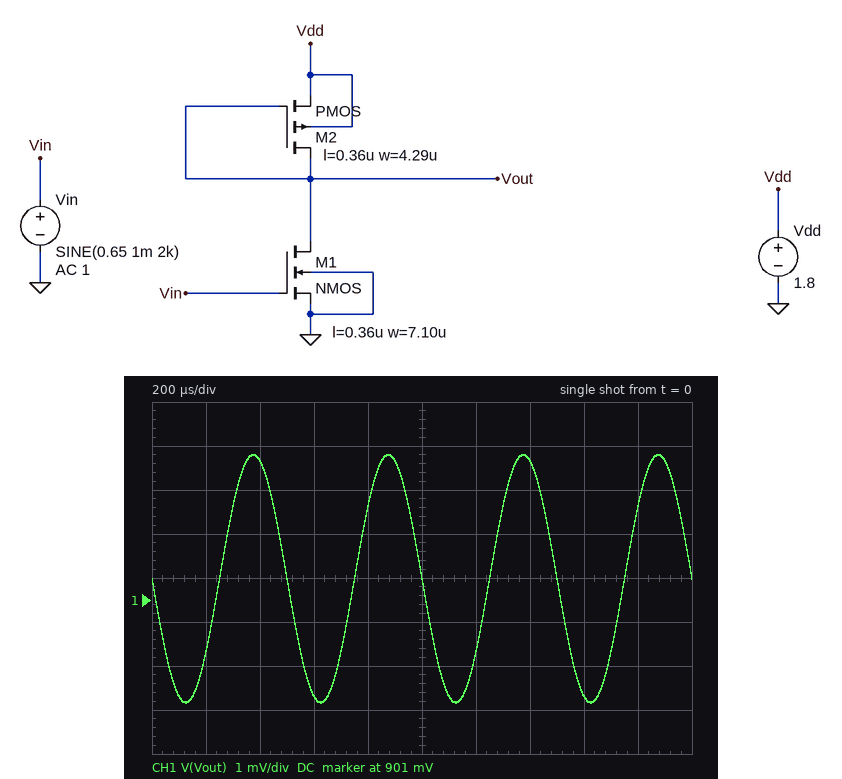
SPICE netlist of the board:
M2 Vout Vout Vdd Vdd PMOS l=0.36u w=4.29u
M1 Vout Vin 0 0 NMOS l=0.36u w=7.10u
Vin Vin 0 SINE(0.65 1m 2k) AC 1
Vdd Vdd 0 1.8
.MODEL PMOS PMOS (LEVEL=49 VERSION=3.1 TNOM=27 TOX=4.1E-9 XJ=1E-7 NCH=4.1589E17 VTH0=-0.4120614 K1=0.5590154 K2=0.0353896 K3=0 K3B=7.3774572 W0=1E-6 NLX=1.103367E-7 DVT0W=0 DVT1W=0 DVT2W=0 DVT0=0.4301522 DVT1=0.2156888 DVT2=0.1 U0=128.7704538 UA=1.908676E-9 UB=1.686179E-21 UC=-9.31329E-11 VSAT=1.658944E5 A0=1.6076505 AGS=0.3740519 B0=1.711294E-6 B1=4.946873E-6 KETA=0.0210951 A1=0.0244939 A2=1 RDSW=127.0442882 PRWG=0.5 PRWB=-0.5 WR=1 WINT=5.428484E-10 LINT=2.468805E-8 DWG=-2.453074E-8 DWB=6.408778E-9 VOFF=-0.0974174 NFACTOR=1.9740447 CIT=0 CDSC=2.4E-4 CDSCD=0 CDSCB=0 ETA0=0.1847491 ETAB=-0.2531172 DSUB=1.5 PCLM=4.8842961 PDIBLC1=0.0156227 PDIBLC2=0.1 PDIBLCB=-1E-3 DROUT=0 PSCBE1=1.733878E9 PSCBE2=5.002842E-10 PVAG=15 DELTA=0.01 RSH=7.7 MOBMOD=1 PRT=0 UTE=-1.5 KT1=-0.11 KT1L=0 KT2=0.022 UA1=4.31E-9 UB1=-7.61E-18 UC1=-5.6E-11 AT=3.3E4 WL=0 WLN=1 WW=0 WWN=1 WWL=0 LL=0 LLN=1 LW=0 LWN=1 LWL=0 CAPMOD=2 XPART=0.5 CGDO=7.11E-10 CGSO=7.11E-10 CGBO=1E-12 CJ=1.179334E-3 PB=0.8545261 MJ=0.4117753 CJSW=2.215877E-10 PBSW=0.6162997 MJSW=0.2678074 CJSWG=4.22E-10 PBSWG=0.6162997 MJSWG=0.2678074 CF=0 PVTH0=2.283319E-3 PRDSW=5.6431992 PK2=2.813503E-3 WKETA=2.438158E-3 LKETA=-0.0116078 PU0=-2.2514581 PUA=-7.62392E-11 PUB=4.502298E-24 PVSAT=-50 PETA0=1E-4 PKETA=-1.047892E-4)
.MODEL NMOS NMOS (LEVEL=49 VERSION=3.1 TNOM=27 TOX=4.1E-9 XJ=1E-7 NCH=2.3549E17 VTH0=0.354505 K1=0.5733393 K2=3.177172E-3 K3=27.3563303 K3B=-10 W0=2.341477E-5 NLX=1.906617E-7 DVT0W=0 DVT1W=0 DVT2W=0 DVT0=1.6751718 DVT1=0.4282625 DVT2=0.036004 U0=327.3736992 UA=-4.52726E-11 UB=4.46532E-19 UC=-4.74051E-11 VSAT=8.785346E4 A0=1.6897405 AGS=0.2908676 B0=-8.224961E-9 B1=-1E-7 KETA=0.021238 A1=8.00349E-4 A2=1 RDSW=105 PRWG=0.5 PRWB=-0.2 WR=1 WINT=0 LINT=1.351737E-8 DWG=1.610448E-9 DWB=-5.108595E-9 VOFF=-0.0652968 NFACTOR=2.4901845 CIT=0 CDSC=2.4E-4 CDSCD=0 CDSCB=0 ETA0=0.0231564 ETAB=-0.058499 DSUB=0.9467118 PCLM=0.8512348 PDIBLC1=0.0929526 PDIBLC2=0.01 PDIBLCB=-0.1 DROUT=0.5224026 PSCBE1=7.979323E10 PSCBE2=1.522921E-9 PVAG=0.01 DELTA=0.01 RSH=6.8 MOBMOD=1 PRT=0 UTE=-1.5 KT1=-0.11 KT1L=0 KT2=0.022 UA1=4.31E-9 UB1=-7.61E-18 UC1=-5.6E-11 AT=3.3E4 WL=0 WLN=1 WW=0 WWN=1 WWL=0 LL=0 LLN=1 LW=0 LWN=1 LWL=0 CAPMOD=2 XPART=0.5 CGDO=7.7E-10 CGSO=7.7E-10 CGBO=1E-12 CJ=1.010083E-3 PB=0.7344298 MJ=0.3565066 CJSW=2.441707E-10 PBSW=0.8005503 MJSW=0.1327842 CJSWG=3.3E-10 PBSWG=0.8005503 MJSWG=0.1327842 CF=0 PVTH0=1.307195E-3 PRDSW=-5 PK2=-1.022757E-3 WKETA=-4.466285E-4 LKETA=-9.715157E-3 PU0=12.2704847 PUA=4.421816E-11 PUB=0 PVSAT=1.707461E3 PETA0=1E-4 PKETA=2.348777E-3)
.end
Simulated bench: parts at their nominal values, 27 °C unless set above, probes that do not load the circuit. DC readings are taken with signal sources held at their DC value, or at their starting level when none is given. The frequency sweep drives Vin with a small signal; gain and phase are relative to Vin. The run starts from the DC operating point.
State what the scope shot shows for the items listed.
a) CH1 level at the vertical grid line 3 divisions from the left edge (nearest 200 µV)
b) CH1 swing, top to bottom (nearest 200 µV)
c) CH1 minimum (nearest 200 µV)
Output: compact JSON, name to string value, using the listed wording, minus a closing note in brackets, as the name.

{"CH1 level at the vertical grid line 3 divisions from the left edge": "898.8 mV", "CH1 swing, top to bottom": "5.6 mV", "CH1 minimum": "898.6 mV"}
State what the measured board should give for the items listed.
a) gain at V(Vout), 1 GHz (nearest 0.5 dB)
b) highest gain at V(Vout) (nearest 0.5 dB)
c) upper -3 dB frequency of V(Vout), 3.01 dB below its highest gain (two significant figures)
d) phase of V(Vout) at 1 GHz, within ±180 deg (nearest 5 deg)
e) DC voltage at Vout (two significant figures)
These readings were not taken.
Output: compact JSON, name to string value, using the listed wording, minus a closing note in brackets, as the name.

{"gain at V(Vout), 1 GHz": "8.5 dB", "highest gain at V(Vout)": "9.0 dB", "upper -3 dB frequency of V(Vout), 3.01 dB below its highest gain": "2.9 GHz", "phase of V(Vout) at 1 GHz, within ±180 deg": "155 deg", "DC voltage at Vout": "900 mV"}
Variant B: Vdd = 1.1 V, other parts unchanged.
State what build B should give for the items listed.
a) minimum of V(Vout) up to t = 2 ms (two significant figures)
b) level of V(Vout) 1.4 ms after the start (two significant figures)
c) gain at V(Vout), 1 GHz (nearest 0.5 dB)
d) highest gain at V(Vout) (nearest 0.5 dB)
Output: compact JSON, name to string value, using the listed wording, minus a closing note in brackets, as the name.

{"minimum of V(Vout) up to t = 2 ms": "220 mV", "level of V(Vout) 1.4 ms after the start": "230 mV", "gain at V(Vout), 1 GHz": "7.5 dB", "highest gain at V(Vout)": "8.0 dB"}
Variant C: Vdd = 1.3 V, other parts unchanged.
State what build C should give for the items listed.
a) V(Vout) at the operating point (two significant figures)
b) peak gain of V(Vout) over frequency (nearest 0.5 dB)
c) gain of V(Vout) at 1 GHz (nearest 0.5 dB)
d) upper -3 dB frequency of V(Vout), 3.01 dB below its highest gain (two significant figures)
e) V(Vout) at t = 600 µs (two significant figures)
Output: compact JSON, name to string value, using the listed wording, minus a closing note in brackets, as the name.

{"V(Vout) at the operating point": "420 mV", "peak gain of V(Vout) over frequency": "8.5 dB", "gain of V(Vout) at 1 GHz": "8.0 dB", "upper -3 dB frequency of V(Vout), 3.01 dB below its highest gain": "2.8 GHz", "V(Vout) at t = 600 µs": "410 mV"}
